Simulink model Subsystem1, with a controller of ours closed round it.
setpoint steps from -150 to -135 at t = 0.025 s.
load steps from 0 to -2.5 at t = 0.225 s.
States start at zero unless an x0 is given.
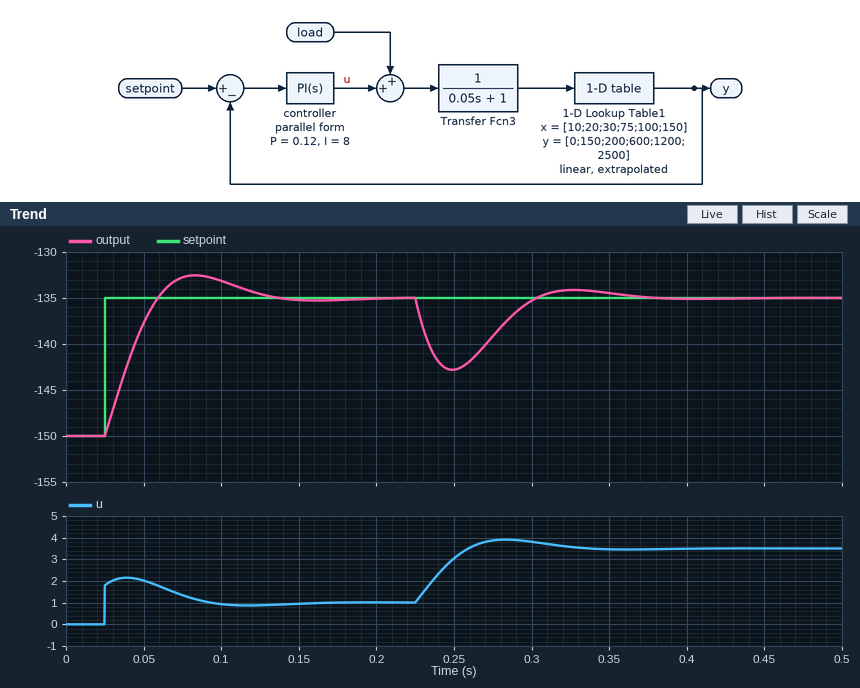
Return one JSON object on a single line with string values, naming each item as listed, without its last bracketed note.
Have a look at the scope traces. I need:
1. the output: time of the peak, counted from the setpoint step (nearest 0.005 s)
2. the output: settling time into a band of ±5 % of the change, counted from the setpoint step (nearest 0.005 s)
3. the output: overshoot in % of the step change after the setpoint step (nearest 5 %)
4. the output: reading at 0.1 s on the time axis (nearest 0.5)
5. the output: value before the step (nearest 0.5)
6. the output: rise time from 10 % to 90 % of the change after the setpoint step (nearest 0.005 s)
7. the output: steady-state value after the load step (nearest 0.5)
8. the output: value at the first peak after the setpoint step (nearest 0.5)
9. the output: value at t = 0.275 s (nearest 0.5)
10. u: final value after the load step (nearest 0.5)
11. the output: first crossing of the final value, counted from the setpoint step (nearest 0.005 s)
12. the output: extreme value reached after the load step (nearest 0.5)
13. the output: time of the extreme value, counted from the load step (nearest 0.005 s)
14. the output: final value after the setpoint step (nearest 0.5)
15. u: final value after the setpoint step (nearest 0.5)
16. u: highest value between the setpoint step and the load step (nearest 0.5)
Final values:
{"the output: time of the peak, counted from the setpoint step": "0.060 s", "the output: settling time into a band of ±5 % of the change, counted from the setpoint step": "0.095 s", "the output: overshoot in % of the step change after the setpoint step": "15 %", "the output: reading at 0.1 s on the time axis": "-133.0", "the output: value before the step": "-150.0", "the output: rise time from 10 % to 90 % of the change after the setpoint step": "0.025 s", "the output: steady-state value after the load step": "-135.0", "the output: value at the first peak after the setpoint step": "-132.5", "the output: value at t = 0.275 s": "-139.0", "u: final value after the load step": "3.5", "the output: first crossing of the final value, counted from the setpoint step": "0.035 s", "the output: extreme value reached after the load step": "-143.0", "the output: time of the extreme value, counted from the load step": "0.025 s", "the output: final value after the setpoint step": "-135.0", "u: final value after the setpoint step": "1.0", "u: highest value between the setpoint step and the load step": "2.0"}
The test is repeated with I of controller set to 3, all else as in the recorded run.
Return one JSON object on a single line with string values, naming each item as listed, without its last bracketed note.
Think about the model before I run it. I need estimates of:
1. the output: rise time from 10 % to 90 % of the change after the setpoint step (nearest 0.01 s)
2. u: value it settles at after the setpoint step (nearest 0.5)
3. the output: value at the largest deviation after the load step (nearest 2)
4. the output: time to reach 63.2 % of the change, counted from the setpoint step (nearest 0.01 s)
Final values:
{"the output: rise time from 10 % to 90 % of the change after the setpoint step": "0.05 s", "u: value it settles at after the setpoint step": "1.0", "the output: value at the largest deviation after the load step": "-144", "the output: time to reach 63.2 % of the change, counted from the setpoint step": "0.03 s"}
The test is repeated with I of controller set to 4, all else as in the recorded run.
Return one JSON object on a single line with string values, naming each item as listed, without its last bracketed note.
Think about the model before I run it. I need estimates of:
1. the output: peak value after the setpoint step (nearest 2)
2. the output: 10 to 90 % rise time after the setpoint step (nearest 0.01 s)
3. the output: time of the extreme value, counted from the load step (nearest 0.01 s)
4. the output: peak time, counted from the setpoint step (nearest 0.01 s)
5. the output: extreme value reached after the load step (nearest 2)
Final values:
{"the output: peak value after the setpoint step": "-134", "the output: 10 to 90 % rise time after the setpoint step": "0.04 s", "the output: time of the extreme value, counted from the load step": "0.03 s", "the output: peak time, counted from the setpoint step": "0.09 s", "the output: extreme value reached after the load step": "-144"}
